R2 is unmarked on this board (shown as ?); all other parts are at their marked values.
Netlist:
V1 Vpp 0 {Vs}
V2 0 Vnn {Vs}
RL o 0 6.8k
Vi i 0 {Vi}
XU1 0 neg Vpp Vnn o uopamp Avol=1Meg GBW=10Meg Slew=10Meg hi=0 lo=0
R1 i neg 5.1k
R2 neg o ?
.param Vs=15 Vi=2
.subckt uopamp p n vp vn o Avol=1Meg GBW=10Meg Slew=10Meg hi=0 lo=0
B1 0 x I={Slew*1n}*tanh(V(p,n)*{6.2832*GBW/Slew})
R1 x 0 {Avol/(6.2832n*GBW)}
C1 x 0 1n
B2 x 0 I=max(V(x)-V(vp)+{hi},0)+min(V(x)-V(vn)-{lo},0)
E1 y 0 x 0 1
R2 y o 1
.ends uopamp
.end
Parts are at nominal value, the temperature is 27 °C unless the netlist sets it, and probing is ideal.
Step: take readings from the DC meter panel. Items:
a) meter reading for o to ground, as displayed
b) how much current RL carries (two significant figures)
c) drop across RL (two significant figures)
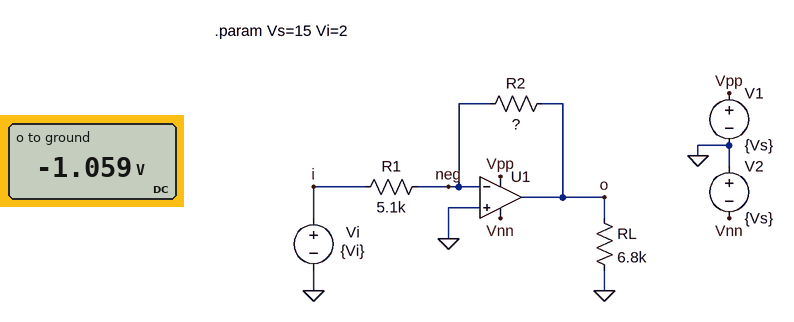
-1.059 V
160 µA
1.1 V
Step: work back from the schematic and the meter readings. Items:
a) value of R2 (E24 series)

2.7 kΩ
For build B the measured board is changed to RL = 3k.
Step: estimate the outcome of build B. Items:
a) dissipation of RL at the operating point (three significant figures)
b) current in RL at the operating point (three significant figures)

374 µW
353 µA
